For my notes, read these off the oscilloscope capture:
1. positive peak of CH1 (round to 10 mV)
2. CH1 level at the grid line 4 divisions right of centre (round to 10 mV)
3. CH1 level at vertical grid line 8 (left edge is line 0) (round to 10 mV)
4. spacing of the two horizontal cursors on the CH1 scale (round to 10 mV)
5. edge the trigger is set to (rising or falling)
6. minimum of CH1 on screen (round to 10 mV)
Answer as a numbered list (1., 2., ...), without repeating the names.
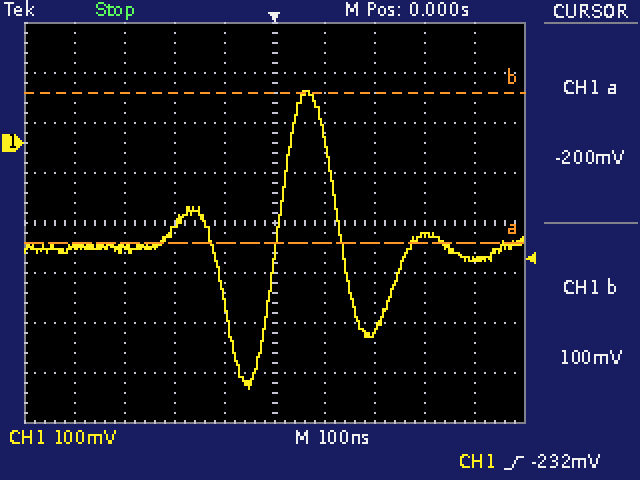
1. 100 mV
2. -230 mV
3. -180 mV
4. 300 mV
5. rising
6. -490 mV
